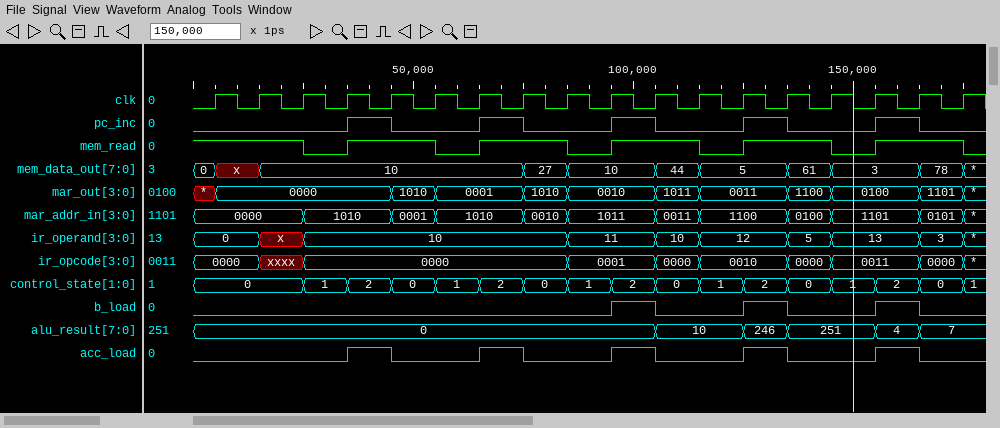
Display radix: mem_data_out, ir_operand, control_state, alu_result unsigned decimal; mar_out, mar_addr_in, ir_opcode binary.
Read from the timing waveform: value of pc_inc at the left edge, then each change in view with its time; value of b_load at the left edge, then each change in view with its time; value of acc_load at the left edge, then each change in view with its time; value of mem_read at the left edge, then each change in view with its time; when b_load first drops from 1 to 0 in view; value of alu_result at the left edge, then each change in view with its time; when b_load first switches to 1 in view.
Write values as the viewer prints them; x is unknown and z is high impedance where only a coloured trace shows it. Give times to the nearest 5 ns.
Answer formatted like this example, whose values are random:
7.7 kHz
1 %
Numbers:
0, 1 at 35 ns, 0 at 45 ns, 1 at 65 ns, 0 at 75 ns, 1 at 95 ns, 0 at 105 ns, 1 at 125 ns, 0 at 135 ns, 1 at 155 ns, 0 at 165 ns
0, 1 at 95 ns, 0 at 105 ns, 1 at 125 ns, 0 at 135 ns, 1 at 155 ns, 0 at 165 ns
0, 1 at 35 ns, 0 at 45 ns, 1 at 65 ns, 0 at 75 ns, 1 at 95 ns, 0 at 105 ns, 1 at 125 ns, 0 at 135 ns, 1 at 155 ns, 0 at 165 ns
1, 0 at 25 ns, 1 at 35 ns, 0 at 55 ns, 1 at 65 ns, 0 at 85 ns, 1 at 95 ns, 0 at 115 ns, 1 at 125 ns, 0 at 145 ns, 1 at 155 ns, 0 at 175 ns
105 ns
0, 10 at 105 ns, 246 at 125 ns, 251 at 135 ns, 4 at 155 ns, 7 at 165 ns
95 ns
